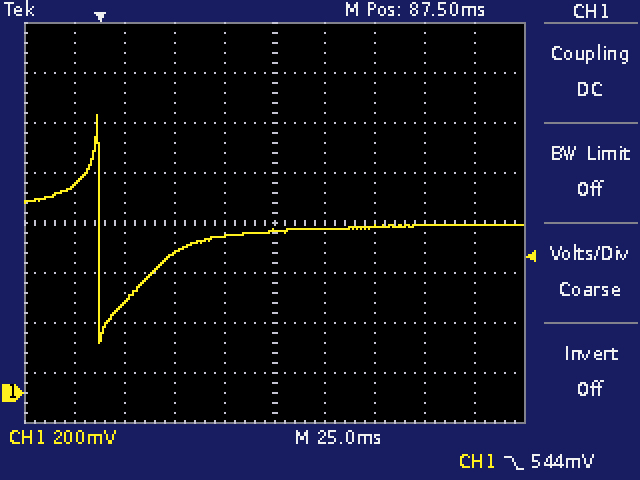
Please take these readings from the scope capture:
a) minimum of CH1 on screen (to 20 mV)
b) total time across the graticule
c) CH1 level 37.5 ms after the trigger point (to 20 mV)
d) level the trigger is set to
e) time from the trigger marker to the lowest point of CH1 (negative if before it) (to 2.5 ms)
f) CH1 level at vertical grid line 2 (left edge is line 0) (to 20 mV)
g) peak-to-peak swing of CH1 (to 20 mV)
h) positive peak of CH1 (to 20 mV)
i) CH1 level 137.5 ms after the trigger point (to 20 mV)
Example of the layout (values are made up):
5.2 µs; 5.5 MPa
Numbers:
200 mV; 250 ms; 560 mV; 544 mV; 0.0 ms; 360 mV; 920 mV; 1.12 V; 660 mV
